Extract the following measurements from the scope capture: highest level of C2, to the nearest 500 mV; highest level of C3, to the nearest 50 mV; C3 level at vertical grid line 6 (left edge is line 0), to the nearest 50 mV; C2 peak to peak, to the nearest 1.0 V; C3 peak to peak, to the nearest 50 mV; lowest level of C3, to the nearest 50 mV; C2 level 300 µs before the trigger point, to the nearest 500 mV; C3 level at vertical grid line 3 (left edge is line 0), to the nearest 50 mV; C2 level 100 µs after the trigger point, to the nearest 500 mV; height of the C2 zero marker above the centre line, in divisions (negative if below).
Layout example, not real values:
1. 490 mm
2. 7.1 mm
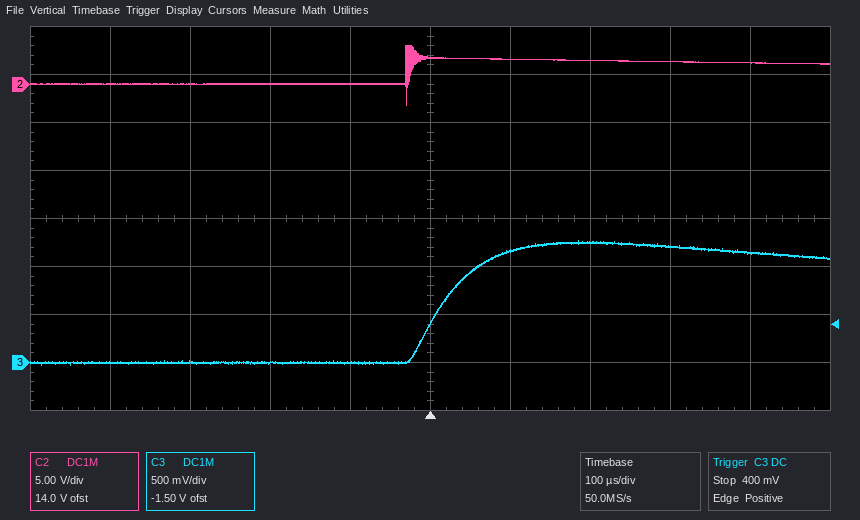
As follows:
1. 4.0 V
2. 1.25 V
3. 1.15 V
4. 6.0 V
5. 1.30 V
6. -50 mV
7. 0.0 V
8. 0 mV
9. 2.5 V
10. +2.8 div
